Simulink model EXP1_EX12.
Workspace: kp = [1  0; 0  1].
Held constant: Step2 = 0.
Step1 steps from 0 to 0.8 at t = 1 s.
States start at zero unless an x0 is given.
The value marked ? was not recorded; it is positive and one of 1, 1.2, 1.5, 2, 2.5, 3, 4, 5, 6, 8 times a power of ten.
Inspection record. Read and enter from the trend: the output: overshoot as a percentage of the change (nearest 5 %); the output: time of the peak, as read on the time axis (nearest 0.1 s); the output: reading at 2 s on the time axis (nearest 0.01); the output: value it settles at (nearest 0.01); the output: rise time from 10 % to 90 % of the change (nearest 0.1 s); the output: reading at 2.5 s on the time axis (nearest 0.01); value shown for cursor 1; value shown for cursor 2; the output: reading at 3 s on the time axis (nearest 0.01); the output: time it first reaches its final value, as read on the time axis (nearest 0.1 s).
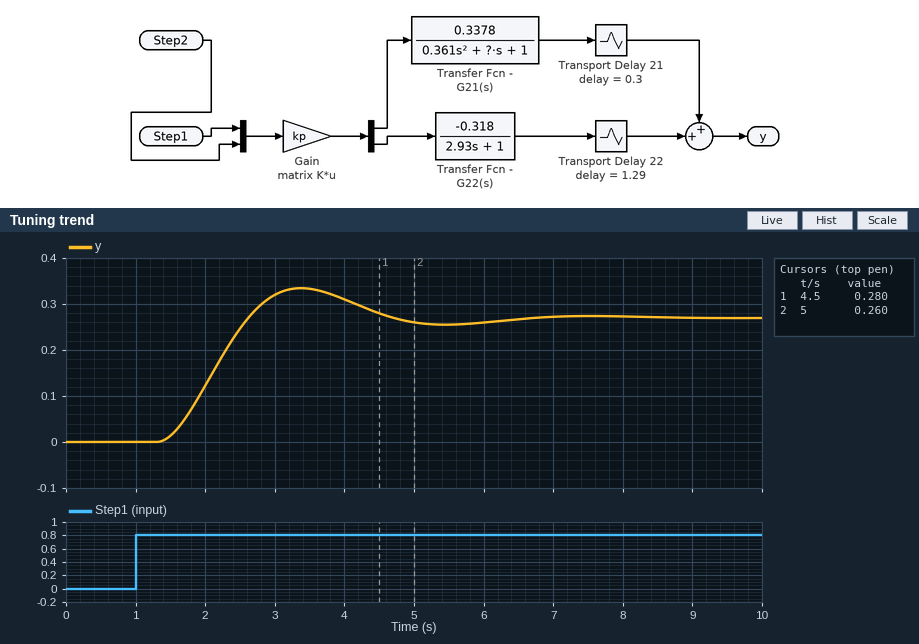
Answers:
25 %
3.4 s
0.12
0.27
0.9 s
0.25
0.280
0.260
0.32
2.6 s
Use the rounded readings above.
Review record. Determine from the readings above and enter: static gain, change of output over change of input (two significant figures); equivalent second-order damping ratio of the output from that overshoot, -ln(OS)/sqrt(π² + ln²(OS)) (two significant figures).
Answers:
0.34
0.40
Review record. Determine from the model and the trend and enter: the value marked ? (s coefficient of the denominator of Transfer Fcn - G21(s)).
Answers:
0.5
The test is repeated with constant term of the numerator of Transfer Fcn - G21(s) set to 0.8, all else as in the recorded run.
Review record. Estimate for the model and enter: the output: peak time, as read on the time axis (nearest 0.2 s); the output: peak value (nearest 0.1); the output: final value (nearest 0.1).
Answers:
3.4 s
0.8
0.6
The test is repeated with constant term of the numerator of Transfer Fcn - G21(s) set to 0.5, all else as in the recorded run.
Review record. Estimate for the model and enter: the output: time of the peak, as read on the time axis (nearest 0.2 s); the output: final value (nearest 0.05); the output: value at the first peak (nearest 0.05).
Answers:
3.4 s
0.40
0.50
